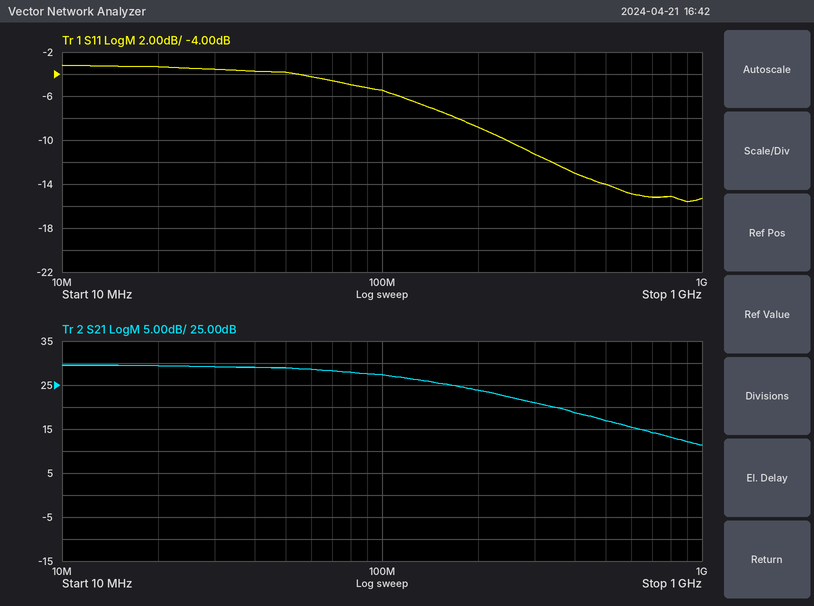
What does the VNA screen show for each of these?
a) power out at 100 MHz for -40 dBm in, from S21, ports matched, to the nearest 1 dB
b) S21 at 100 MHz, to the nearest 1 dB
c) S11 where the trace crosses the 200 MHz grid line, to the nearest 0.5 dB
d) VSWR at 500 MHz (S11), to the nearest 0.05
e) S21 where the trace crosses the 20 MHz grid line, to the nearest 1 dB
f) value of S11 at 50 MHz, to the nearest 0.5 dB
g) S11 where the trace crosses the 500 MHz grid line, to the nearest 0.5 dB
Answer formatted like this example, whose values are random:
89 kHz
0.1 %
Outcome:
-13 dBm
27 dB
-9.0 dB
1.50
29 dB
-4.0 dB
-14.0 dB
